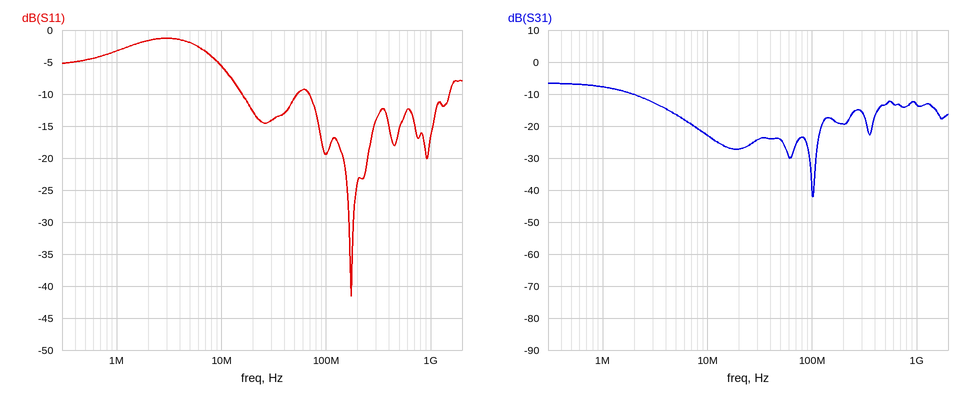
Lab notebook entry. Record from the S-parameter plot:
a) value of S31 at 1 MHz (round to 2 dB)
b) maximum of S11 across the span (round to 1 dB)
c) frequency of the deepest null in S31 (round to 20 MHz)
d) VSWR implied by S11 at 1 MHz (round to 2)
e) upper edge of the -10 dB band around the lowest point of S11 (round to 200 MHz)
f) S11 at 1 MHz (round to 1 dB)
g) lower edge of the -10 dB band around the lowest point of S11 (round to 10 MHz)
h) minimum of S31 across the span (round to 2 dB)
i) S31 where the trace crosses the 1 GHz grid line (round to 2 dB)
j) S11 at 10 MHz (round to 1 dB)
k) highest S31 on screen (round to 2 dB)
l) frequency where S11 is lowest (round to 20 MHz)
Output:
-8 dB
-1 dB
100 MHz
6
1.6 GHz
-3 dB
70 MHz
-42 dB
-14 dB
-6 dB
-6 dB
180 MHz
